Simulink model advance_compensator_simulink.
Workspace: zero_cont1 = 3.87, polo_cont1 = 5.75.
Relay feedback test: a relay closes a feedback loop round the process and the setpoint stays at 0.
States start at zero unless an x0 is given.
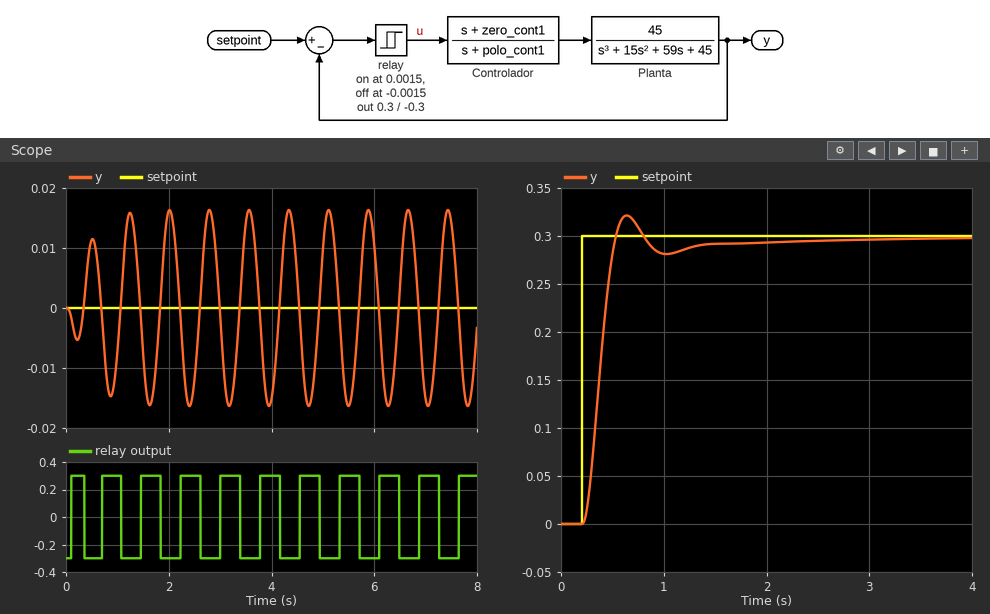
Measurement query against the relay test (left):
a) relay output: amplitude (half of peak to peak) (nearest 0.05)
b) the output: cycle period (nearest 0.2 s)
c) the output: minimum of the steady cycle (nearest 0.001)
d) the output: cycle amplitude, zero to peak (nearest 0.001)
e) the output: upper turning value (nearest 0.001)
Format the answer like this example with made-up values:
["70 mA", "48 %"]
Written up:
["0.30", "0.8 s", "-0.016", "0.016", "0.016"]
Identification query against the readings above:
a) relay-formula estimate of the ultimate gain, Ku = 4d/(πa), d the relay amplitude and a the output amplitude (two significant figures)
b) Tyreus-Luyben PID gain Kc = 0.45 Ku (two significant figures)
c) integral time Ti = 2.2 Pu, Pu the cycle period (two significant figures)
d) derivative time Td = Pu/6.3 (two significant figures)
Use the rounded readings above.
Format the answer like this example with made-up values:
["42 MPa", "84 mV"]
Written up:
["24", "11", "1.8 s", "0.13 s"]
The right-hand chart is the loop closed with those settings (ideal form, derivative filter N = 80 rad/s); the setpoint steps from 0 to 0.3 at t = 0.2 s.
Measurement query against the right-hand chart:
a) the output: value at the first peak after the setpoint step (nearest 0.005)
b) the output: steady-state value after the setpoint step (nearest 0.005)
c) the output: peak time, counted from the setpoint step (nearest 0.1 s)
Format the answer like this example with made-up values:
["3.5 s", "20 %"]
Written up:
["0.320", "0.300", "0.4 s"]
